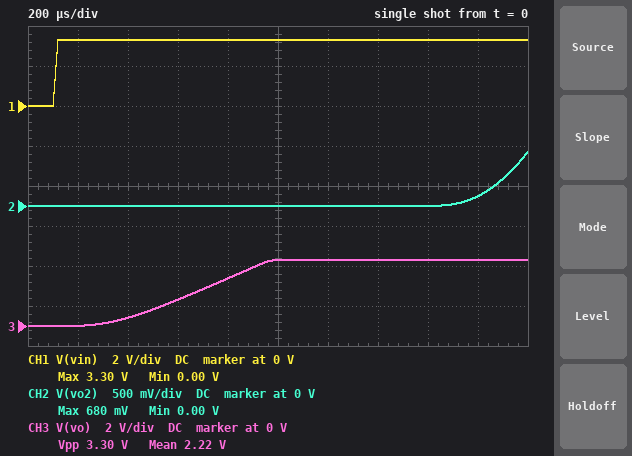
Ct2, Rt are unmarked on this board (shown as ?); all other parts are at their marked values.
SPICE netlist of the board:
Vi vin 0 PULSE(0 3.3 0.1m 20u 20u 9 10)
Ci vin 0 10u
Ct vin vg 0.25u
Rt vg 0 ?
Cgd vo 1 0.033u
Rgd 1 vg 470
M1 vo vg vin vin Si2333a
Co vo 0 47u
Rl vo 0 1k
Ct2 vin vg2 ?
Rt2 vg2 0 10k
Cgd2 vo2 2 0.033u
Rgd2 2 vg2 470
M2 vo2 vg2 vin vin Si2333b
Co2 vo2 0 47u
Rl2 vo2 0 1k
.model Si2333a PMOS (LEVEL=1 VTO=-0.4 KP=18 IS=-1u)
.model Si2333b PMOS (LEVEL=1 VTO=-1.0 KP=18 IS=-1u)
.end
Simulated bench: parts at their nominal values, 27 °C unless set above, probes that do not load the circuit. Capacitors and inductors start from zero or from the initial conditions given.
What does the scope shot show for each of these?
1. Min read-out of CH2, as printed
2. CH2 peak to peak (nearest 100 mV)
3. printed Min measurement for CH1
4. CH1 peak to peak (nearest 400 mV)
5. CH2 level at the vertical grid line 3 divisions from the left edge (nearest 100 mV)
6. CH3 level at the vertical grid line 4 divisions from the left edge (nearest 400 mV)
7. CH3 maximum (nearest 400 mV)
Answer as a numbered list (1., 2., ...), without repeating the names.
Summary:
1. 0.00 V
2. 700 mV
3. 0.00 V
4. 3.2 V
5. 0 V
6. 2.4 V
7. 3.2 V
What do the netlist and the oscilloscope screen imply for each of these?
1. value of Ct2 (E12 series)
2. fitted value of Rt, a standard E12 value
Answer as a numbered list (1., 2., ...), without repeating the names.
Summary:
1. 470 nF
2. 15 kΩ
